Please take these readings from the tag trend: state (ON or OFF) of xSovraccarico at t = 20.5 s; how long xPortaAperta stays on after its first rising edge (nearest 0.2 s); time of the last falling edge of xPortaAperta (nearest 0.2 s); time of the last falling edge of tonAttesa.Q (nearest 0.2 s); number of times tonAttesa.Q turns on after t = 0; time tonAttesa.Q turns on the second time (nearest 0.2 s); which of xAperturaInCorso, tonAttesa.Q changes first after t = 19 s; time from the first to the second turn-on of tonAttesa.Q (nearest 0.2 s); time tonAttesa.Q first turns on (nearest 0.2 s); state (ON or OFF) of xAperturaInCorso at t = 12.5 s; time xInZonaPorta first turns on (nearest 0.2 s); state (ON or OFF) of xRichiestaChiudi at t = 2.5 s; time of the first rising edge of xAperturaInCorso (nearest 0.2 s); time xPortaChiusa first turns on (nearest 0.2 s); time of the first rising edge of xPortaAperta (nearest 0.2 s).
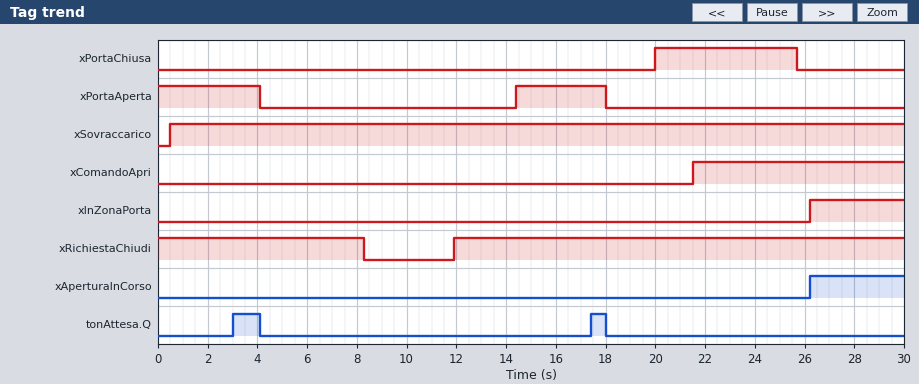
ON
3.6 s
18.0 s
18.0 s
2
17.4 s
xAperturaInCorso
14.4 s
3.0 s
OFF
26.2 s
ON
26.2 s
20.0 s
14.4 s
